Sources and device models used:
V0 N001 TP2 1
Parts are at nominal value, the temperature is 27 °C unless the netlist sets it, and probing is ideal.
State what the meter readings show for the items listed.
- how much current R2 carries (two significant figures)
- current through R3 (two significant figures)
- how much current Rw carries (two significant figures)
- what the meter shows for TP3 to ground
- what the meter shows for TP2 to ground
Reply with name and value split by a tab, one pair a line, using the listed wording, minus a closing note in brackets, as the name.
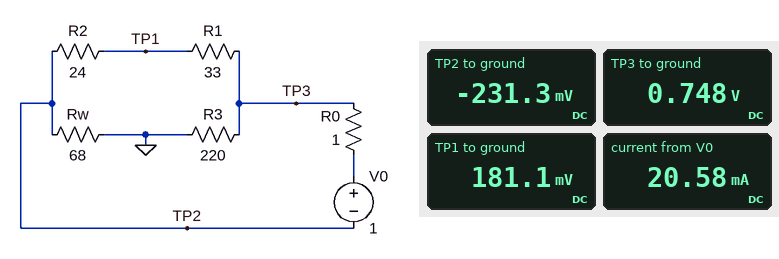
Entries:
how much current R2 carries	17 mA
current through R3	3.4 mA
how much current Rw carries	3.4 mA
what the meter shows for TP3 to ground	0.748 V
what the meter shows for TP2 to ground	-231.3 mV
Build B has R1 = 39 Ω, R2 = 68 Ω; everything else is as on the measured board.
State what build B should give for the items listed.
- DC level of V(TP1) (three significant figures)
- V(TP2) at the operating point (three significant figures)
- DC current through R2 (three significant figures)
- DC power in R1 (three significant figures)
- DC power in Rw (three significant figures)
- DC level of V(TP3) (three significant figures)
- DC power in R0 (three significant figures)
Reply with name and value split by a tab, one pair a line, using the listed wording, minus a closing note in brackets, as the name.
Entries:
DC level of V(TP1)	394 mV
V(TP2) at the operating point	-233 mV
DC current through R2	9.23 mA
DC power in R1	3.32 mW
DC power in Rw	799 µW
DC level of V(TP3)	754 mV
DC power in R0	160 µW
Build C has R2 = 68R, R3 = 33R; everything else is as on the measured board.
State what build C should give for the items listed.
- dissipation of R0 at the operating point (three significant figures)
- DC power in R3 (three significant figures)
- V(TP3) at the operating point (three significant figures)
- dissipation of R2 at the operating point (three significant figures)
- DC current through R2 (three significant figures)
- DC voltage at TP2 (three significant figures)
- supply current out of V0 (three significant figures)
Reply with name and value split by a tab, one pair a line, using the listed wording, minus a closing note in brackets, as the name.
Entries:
dissipation of R0 at the operating point	377 µW
DC power in R3	3.11 mW
V(TP3) at the operating point	320 mV
dissipation of R2 at the operating point	6.41 mW
DC current through R2	9.71 mA
DC voltage at TP2	-660 mV
supply current out of V0	19.4 mA
